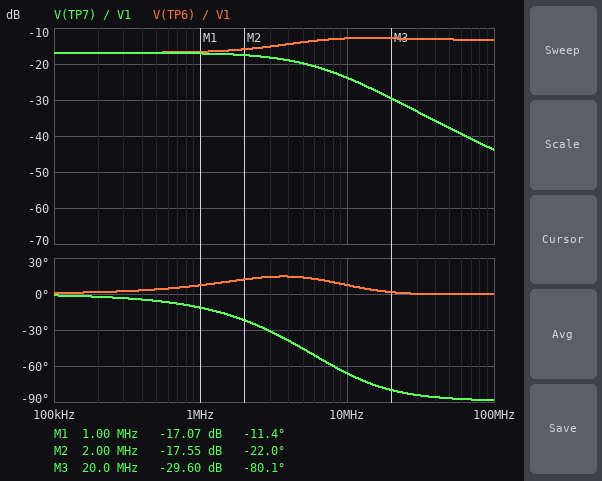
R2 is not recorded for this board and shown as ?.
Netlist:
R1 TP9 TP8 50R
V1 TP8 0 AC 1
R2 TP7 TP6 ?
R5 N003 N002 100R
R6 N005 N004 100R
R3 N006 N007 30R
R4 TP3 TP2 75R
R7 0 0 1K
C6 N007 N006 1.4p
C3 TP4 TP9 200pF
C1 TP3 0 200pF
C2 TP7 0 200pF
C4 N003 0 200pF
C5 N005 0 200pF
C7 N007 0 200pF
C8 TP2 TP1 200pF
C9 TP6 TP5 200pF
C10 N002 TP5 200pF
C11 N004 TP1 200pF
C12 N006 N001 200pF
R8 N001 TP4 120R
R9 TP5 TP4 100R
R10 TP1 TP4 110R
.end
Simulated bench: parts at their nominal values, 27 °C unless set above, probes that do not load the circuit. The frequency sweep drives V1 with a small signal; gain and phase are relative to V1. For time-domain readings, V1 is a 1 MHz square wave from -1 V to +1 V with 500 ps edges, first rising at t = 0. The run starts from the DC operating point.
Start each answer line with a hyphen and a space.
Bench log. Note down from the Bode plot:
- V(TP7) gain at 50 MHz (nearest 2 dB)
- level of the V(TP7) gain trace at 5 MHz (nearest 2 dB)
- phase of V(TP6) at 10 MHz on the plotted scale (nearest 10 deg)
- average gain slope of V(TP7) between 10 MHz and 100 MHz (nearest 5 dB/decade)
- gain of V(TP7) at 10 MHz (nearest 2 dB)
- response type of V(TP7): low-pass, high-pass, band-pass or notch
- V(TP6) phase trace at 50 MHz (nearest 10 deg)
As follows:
- -38 dB
- -20 dB
- 10 deg
- -20 dB/decade
- -24 dB
- low-pass
- 0 deg
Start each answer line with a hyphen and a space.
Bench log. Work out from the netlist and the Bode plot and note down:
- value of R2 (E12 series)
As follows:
- 270 Ω
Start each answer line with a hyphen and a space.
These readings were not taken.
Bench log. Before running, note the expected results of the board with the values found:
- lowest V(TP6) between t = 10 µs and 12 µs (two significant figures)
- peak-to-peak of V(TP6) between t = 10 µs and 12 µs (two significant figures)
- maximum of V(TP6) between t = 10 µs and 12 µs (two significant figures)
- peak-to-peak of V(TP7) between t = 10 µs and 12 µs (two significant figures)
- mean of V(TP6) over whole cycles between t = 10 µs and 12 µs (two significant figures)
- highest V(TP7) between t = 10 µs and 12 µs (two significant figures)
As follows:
- -150 mV
- 580 mV
- 430 mV
- 290 mV
- 140 mV
- 290 mV
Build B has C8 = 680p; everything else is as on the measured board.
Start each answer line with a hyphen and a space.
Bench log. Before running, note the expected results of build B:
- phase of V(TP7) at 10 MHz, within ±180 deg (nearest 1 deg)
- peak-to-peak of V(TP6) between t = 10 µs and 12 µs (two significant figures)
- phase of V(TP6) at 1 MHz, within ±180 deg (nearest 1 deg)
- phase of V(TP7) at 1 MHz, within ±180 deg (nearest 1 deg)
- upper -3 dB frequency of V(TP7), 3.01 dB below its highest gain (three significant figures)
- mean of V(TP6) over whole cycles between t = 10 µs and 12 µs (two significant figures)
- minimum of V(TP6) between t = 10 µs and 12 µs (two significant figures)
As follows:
- -65 deg
- 600 mV
- 8 deg
- -10 deg
- 5.68 MHz
- 130 mV
- -170 mV
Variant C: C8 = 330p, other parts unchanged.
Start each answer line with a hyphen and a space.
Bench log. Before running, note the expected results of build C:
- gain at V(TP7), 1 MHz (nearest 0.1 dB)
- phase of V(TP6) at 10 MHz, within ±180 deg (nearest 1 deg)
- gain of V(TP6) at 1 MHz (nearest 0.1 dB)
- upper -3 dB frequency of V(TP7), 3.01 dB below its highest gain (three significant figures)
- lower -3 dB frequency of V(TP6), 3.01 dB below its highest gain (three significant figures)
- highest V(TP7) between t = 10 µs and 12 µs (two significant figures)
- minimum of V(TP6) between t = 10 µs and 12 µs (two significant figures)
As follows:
- -17.4 dB
- 8 deg
- -16.9 dB
- 5.33 MHz
- 2.41 MHz
- 280 mV
- -160 mV
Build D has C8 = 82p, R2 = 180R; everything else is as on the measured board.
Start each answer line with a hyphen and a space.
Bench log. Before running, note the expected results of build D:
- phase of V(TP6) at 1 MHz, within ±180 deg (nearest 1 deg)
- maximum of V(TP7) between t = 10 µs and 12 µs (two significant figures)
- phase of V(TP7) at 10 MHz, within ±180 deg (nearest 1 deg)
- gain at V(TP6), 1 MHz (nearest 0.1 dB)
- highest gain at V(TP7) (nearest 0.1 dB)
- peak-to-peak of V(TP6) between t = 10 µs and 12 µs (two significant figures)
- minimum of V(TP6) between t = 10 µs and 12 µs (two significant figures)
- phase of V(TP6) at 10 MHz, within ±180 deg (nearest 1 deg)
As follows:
- 3 deg
- 300 mV
- -59 deg
- -16.3 dB
- -16.4 dB
- 490 mV
- -94 mV
- 7 deg
